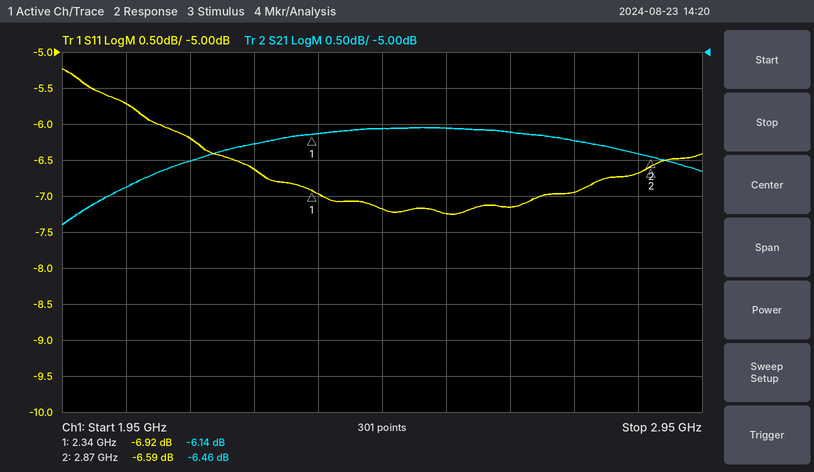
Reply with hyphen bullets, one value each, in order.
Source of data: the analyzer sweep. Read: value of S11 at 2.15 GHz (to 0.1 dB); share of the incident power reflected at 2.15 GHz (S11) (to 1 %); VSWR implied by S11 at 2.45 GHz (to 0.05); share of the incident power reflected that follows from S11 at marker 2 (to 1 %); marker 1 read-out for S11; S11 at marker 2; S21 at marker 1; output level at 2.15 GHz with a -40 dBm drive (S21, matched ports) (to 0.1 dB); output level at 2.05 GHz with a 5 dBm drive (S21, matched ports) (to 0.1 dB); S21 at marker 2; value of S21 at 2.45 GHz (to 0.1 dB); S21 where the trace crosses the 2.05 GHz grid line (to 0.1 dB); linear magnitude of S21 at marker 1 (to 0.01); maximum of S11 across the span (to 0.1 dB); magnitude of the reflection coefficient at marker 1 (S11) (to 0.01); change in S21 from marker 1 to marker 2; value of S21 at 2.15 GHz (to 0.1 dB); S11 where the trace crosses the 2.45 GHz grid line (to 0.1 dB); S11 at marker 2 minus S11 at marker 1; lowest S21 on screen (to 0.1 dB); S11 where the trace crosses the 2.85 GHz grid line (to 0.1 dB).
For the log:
- -6.2 dB
- 24 %
- 2.55
- 22 %
- -6.92 dB
- -6.59 dB
- -6.14 dB
- -46.5 dBm
- -1.9 dBm
- -6.46 dB
- -6.1 dB
- -6.9 dB
- 0.49
- -5.2 dB
- 0.45
- -0.32 dB
- -6.5 dB
- -7.2 dB
- 0.33 dB
- -7.4 dB
- -6.7 dB
